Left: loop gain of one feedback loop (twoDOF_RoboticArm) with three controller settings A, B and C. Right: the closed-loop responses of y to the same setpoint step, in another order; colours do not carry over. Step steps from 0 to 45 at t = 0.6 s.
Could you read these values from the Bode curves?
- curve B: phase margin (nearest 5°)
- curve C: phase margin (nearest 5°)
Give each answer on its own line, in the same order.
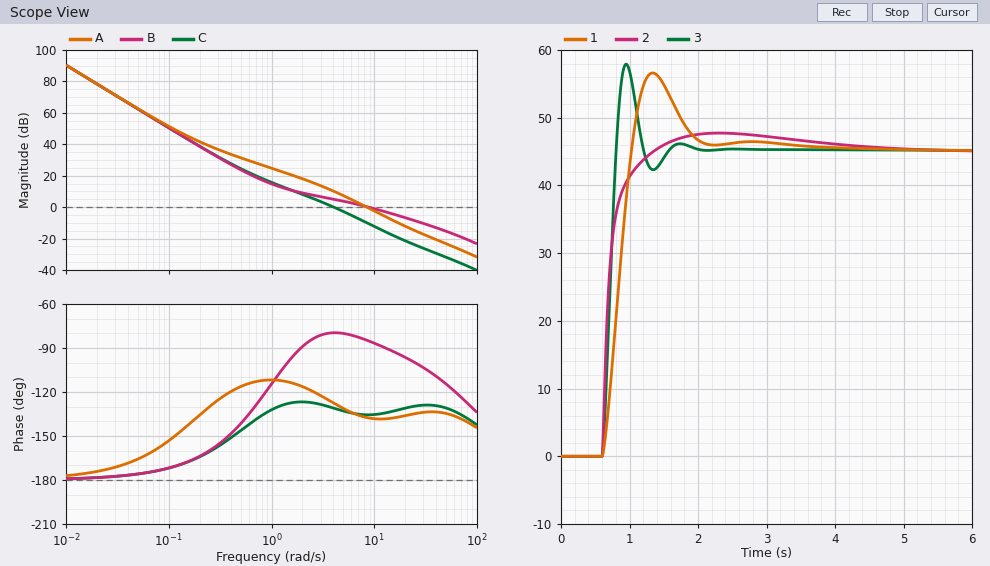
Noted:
95°
50°
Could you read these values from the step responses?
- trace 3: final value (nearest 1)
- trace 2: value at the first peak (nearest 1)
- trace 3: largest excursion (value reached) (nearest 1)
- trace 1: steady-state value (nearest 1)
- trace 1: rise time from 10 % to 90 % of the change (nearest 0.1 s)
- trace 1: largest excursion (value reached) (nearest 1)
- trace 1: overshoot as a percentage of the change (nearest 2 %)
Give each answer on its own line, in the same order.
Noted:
45
48
58
45
0.3 s
57
26 %
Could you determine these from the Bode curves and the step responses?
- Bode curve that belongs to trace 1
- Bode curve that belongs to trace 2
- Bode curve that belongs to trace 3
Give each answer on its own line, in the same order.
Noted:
C
B
A
